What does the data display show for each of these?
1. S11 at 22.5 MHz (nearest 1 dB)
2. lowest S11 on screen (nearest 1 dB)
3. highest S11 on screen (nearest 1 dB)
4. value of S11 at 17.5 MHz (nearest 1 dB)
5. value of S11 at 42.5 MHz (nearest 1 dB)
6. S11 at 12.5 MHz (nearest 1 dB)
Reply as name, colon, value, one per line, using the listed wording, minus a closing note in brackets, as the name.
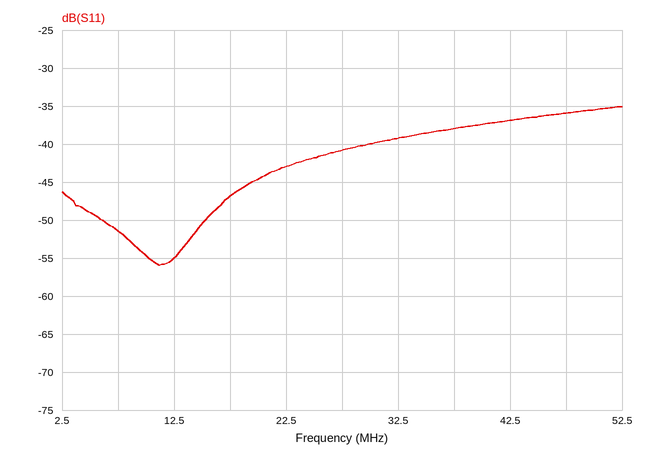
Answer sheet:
S11 at 22.5 MHz: -43 dB
lowest S11 on screen: -56 dB
highest S11 on screen: -35 dB
value of S11 at 17.5 MHz: -47 dB
value of S11 at 42.5 MHz: -37 dB
S11 at 12.5 MHz: -55 dB
